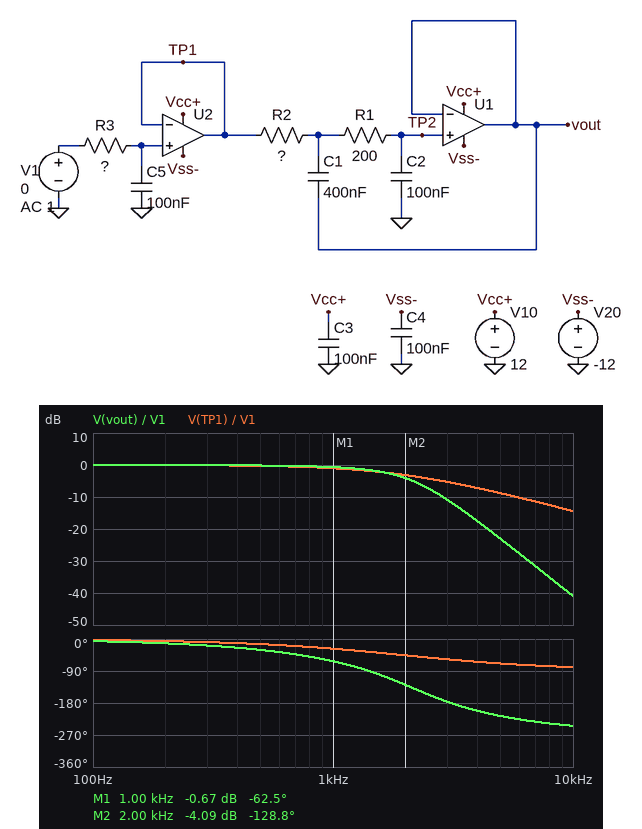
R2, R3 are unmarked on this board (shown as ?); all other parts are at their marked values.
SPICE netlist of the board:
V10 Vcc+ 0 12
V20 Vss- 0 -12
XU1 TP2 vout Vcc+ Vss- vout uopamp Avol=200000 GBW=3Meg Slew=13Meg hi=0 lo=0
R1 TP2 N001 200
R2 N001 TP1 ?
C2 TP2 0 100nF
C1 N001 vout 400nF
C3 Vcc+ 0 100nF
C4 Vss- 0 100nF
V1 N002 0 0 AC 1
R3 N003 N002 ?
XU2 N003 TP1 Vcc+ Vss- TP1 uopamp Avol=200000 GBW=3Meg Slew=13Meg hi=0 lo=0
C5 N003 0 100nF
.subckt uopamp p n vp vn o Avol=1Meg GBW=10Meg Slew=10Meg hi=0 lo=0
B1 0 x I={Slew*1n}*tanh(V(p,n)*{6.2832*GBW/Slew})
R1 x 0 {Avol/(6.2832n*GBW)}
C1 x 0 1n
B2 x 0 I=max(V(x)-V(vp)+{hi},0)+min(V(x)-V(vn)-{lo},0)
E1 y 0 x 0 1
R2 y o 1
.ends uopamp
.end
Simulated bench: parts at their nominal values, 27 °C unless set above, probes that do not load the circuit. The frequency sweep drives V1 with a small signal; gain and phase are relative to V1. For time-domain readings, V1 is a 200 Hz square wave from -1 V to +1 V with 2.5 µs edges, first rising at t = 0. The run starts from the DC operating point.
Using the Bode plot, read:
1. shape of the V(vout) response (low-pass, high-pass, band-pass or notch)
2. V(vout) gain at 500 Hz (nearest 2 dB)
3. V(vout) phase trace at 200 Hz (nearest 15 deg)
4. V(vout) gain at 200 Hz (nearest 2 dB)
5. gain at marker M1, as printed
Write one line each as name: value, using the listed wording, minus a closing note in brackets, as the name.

shape of the V(vout) response: low-pass
V(vout) gain at 500 Hz: 0 dB
V(vout) phase trace at 200 Hz: -15 deg
V(vout) gain at 200 Hz: 0 dB
gain at marker M1, as printed: -0.67 dB
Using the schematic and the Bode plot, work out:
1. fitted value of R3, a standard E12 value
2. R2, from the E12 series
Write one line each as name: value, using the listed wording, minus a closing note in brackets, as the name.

fitted value of R3, a standard E12 value: 820 Ω
R2, from the E12 series: 680 Ω
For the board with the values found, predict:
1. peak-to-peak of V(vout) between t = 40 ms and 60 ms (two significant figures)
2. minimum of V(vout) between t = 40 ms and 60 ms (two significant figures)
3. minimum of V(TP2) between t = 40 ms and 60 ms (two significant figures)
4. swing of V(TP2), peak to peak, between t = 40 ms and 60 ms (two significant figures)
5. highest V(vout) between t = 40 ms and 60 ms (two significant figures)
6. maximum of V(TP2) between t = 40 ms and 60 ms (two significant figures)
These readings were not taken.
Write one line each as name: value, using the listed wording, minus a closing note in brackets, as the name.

peak-to-peak of V(vout) between t = 40 ms and 60 ms: 2.1 V
minimum of V(vout) between t = 40 ms and 60 ms: -1.1 V
minimum of V(TP2) between t = 40 ms and 60 ms: -1.1 V
swing of V(TP2), peak to peak, between t = 40 ms and 60 ms: 2.1 V
highest V(vout) between t = 40 ms and 60 ms: 1.1 V
maximum of V(TP2) between t = 40 ms and 60 ms: 1.1 V
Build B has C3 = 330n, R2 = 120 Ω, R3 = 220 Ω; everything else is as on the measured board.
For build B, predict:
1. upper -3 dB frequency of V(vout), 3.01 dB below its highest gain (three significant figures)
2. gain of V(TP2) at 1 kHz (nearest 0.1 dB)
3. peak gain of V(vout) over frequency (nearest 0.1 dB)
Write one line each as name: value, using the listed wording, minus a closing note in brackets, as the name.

upper -3 dB frequency of V(vout), 3.01 dB below its highest gain: 5.41 kHz
gain of V(TP2) at 1 kHz: 0.1 dB
peak gain of V(vout) over frequency: 0.3 dB
